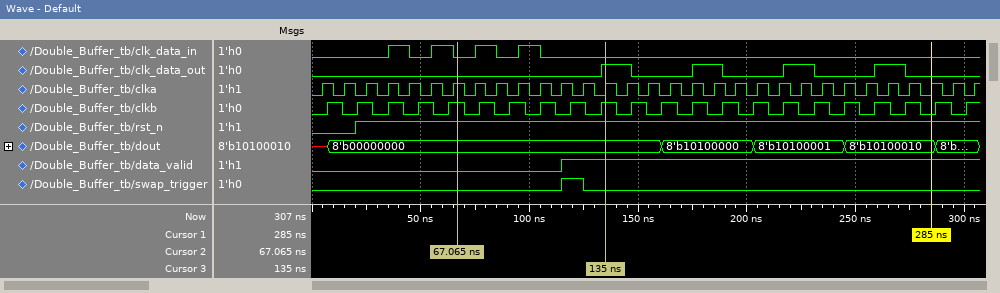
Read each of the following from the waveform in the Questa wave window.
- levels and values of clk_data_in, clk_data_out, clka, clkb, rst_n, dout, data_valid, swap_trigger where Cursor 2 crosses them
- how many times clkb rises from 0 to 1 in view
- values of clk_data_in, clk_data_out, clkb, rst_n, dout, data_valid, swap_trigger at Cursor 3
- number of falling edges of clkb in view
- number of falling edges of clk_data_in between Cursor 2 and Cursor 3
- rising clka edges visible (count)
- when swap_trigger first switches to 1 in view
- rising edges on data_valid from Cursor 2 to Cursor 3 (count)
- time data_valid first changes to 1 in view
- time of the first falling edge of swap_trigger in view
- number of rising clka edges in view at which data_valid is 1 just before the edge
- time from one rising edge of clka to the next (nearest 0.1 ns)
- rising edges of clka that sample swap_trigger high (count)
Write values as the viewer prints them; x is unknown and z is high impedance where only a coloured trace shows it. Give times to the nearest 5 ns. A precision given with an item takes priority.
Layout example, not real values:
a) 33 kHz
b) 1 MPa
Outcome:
a) clk_data_in=0, clk_data_out=0, clka=1, clkb=1, rst_n=1, dout=8'b00000000, data_valid=0, swap_trigger=0
b) 22
c) clk_data_in=0, clk_data_out=1, clkb=1, rst_n=1, dout=8'b00000000, data_valid=1, swap_trigger=0
d) 21
e) 2
f) 31
g) 115 ns
h) 1
i) 115 ns
j) 125 ns
k) 19
l) 10 ns
m) 1
